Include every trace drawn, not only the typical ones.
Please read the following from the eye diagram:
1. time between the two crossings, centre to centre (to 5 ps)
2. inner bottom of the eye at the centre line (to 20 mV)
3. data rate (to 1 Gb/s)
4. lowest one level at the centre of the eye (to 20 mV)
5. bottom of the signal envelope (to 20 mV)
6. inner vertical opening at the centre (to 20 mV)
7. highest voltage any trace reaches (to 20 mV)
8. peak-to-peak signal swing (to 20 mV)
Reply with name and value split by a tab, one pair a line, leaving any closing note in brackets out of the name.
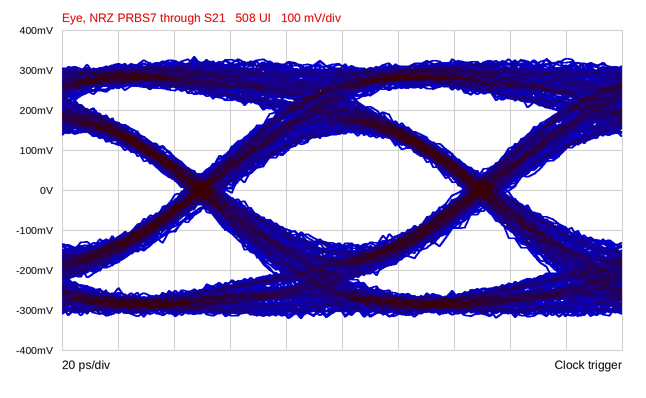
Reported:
time between the two crossings, centre to centre	100 ps
inner bottom of the eye at the centre line	-140 mV
data rate	10 Gb/s
lowest one level at the centre of the eye	140 mV
bottom of the signal envelope	-320 mV
inner vertical opening at the centre	280 mV
highest voltage any trace reaches	340 mV
peak-to-peak signal swing	660 mV
